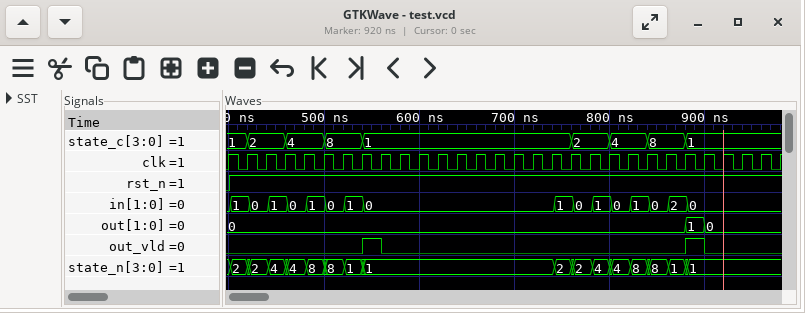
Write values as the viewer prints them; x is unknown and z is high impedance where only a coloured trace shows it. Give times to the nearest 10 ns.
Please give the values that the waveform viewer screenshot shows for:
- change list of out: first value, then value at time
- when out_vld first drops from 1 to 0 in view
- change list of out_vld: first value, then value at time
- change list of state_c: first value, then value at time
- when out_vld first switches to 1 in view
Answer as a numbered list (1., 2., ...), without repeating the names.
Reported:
1. 0, 1 at 880 ns, 0 at 900 ns
2. 560 ns
3. 0, 1 at 540 ns, 0 at 560 ns, 1 at 880 ns, 0 at 900 ns
4. 1, 2 at 420 ns, 4 at 460 ns, 8 at 500 ns, 1 at 540 ns, 2 at 760 ns, 4 at 800 ns, 8 at 840 ns, 1 at 880 ns
5. 540 ns
